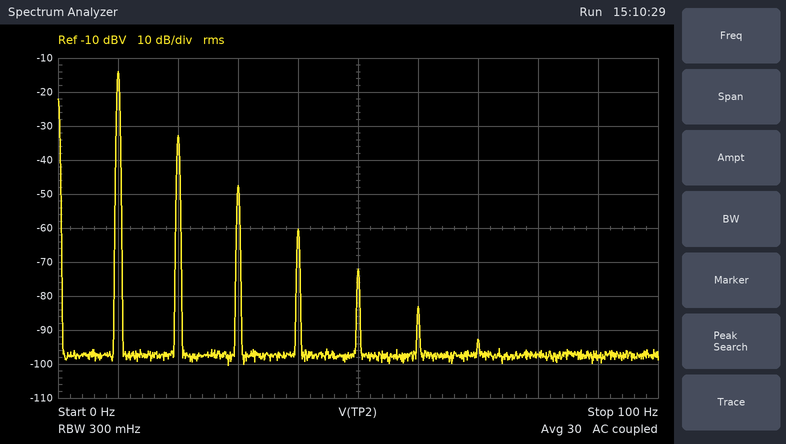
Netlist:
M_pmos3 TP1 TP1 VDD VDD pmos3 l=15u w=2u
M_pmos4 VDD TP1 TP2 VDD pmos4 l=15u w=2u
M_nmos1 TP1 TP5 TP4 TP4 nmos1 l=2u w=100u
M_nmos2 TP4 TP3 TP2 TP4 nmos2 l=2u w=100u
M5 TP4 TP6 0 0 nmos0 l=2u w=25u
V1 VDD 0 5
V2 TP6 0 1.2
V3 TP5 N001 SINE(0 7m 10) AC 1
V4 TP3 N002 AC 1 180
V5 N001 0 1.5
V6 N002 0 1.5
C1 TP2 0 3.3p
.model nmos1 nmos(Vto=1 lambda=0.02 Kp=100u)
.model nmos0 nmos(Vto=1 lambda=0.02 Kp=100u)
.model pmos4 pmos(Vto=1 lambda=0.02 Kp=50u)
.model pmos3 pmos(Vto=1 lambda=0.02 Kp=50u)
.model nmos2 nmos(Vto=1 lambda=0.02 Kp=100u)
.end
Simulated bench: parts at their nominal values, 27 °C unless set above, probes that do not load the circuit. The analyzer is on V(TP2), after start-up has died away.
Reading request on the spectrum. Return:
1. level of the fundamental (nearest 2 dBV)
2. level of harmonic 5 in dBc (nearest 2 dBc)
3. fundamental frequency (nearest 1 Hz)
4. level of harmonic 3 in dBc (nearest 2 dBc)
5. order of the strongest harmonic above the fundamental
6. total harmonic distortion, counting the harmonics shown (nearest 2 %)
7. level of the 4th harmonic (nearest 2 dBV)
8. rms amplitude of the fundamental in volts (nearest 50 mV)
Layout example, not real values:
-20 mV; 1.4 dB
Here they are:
-14 dBV; -58 dBc; 10 Hz; -34 dBc; 2; 12 %; -60 dBV; 200 mV
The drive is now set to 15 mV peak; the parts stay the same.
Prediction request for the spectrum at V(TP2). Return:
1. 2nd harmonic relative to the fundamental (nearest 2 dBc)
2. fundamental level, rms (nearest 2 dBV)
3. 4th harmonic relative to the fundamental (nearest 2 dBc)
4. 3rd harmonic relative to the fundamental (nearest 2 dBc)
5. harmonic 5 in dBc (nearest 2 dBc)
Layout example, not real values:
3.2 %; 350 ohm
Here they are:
-6 dBc; 0 dBV; -18 dBc; -10 dBc; -34 dBc
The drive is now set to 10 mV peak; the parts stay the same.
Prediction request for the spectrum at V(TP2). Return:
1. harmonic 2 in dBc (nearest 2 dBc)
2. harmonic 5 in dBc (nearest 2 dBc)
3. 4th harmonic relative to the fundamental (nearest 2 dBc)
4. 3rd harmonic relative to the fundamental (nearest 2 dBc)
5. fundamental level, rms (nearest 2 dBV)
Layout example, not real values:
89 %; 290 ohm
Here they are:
-14 dBc; -38 dBc; -32 dBc; -24 dBc; -10 dBV
